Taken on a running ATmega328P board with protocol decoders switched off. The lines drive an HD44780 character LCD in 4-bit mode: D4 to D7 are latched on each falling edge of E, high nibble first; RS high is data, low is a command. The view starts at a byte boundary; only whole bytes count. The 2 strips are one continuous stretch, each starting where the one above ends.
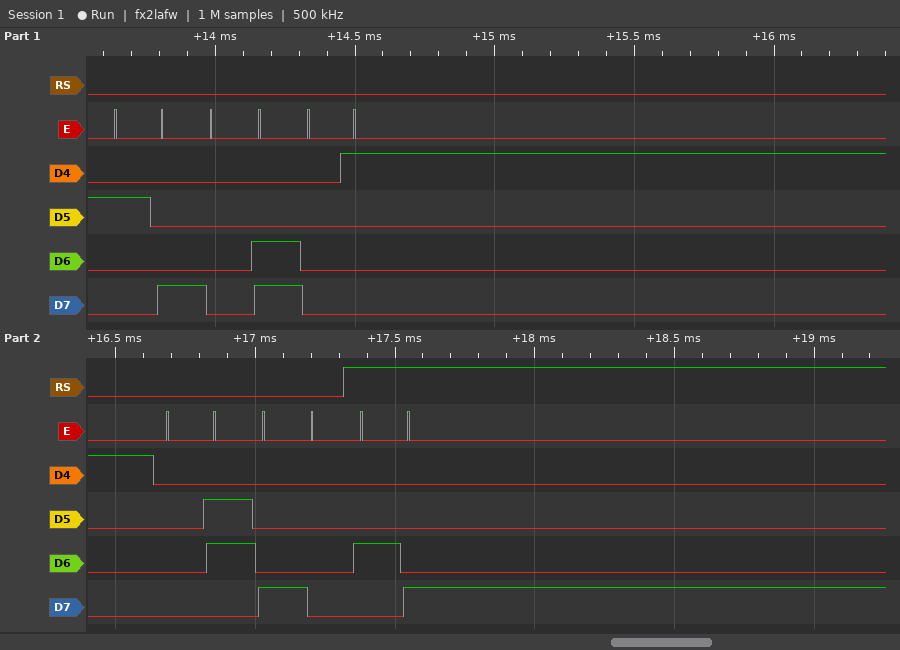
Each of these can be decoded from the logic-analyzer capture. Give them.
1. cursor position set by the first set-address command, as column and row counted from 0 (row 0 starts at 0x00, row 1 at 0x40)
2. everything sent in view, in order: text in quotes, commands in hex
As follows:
column 0, row 0
0x28 0x0C 0x01 0x06 0x80 "H"
